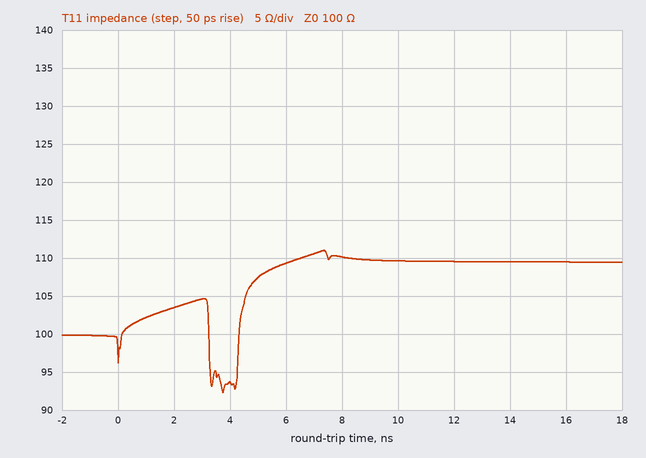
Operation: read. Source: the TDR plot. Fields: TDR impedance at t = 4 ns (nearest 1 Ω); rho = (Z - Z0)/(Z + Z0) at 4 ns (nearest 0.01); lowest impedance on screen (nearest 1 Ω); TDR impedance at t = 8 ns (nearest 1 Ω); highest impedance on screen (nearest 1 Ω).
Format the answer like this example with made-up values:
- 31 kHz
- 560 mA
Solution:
- 94 Ω
- -0.03
- 92 Ω
- 110 Ω
- 111 Ω
